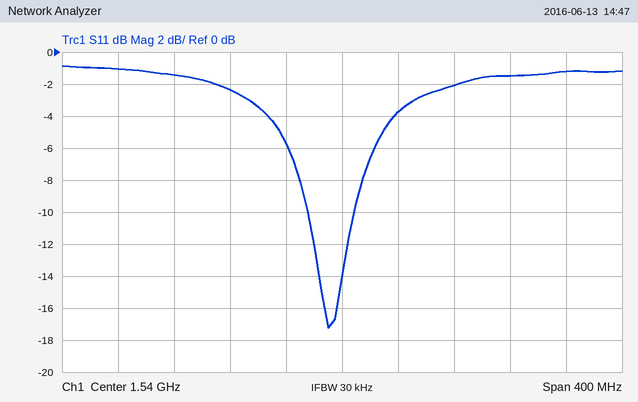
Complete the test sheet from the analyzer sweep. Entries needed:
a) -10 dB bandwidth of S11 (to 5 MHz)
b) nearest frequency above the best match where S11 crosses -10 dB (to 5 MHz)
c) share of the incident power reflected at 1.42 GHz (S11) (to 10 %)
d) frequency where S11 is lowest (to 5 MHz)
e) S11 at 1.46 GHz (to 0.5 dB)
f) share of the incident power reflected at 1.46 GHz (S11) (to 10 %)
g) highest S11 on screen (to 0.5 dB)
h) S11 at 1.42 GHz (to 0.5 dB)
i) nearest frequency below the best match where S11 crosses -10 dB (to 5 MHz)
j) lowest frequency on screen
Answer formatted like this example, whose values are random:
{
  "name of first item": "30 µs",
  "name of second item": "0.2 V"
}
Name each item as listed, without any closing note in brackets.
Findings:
{
  "-10 dB bandwidth of S11": "35 MHz",
  "nearest frequency above the best match where S11 crosses -10 dB": "1.550 GHz",
  "share of the incident power reflected at 1.42 GHz (S11)": "70 %",
  "frequency where S11 is lowest": "1.530 GHz",
  "S11 at 1.46 GHz": "-2.5 dB",
  "share of the incident power reflected at 1.46 GHz (S11)": "60 %",
  "highest S11 on screen": "-1.0 dB",
  "S11 at 1.42 GHz": "-1.5 dB",
  "nearest frequency below the best match where S11 crosses -10 dB": "1.515 GHz",
  "lowest frequency on screen": "1.34 GHz"
}
